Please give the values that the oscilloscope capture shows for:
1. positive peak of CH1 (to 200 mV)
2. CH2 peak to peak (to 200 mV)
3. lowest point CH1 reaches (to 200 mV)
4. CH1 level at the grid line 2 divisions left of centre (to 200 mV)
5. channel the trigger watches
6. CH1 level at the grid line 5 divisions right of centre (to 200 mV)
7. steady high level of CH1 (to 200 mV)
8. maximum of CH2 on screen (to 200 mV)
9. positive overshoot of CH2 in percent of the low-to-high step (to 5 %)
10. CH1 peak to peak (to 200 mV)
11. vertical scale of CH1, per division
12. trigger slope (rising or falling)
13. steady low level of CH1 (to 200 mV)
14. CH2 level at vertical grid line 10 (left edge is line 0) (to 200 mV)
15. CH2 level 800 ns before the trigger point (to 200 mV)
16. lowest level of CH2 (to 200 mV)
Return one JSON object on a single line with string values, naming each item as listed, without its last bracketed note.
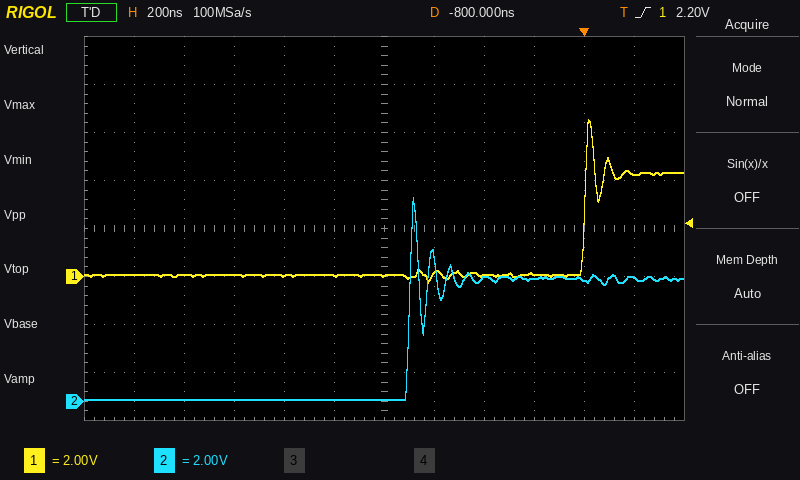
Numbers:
{"positive peak of CH1": "6.6 V", "CH2 peak to peak": "8.4 V", "lowest point CH1 reaches": "-200 mV", "CH1 level at the grid line 2 divisions left of centre": "0.0 V", "channel the trigger watches": "CH1", "CH1 level at the grid line 5 divisions right of centre": "4.2 V", "steady high level of CH1": "4.4 V", "maximum of CH2 on screen": "8.4 V", "positive overshoot of CH2 in percent of the low-to-high step": "65 %", "CH1 peak to peak": "6.8 V", "vertical scale of CH1, per division": "2 V", "trigger slope": "rising", "steady low level of CH1": "0.0 V", "CH2 level at vertical grid line 10 (left edge is line 0)": "5.0 V", "CH2 level 800 ns before the trigger point": "0.0 V", "lowest level of CH2": "0.0 V"}
